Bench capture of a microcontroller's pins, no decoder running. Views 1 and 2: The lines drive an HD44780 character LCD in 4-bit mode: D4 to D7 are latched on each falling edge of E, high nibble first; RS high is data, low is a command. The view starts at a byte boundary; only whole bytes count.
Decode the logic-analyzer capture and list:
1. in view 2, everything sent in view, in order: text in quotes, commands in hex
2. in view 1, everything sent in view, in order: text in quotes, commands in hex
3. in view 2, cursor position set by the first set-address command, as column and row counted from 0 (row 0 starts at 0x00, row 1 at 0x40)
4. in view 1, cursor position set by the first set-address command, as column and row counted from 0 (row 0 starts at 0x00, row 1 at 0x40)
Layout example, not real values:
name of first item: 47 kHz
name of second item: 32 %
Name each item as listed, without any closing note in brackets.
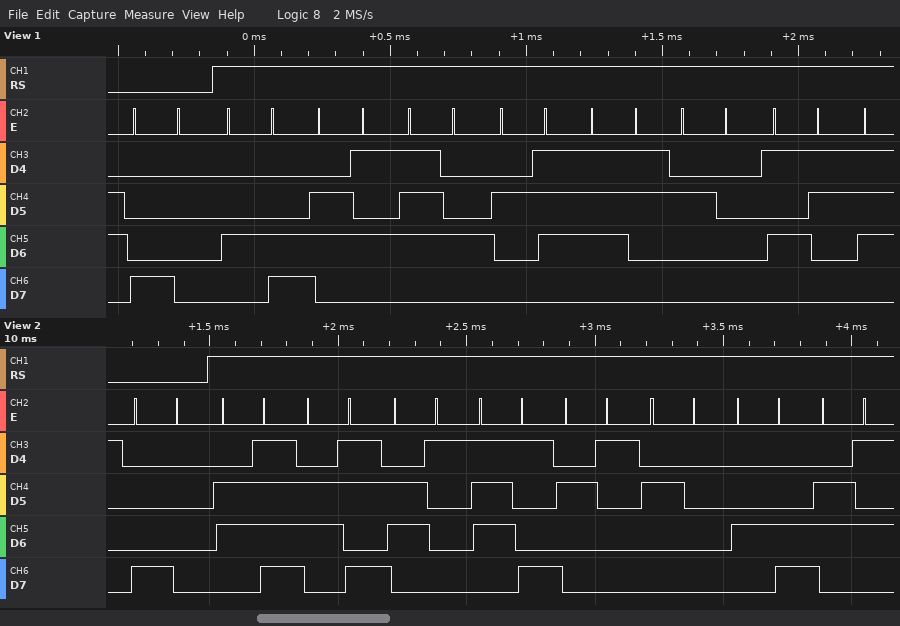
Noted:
in view 2, everything sent in view, in order: text in quotes, commands in hex: 0x80 "okay! Le"
in view 1, everything sent in view, in order: text in quotes, commands in hex: 0x80 "Let's S"
in view 2, cursor position set by the first set-address command, as column and row counted from 0: column 0, row 0
in view 1, cursor position set by the first set-address command, as column and row counted from 0: column 0, row 0
